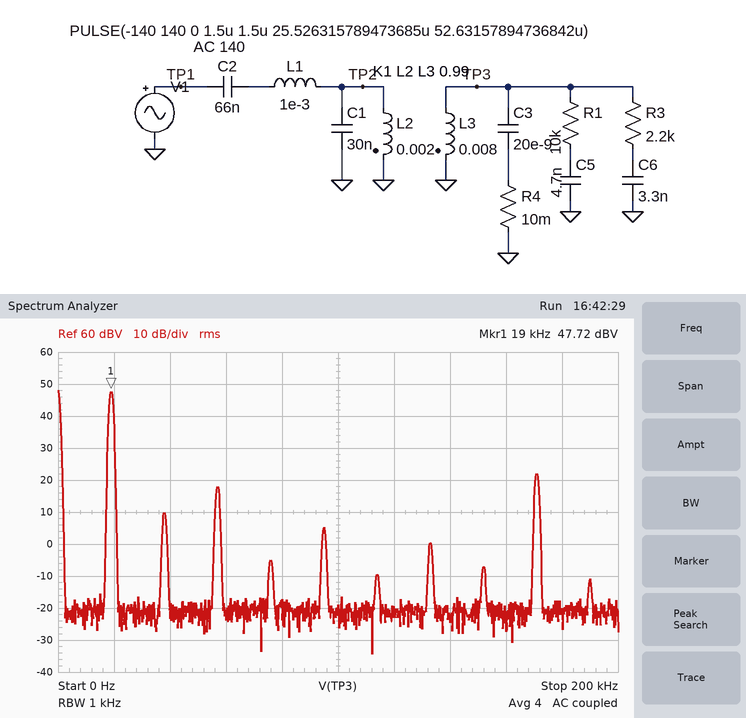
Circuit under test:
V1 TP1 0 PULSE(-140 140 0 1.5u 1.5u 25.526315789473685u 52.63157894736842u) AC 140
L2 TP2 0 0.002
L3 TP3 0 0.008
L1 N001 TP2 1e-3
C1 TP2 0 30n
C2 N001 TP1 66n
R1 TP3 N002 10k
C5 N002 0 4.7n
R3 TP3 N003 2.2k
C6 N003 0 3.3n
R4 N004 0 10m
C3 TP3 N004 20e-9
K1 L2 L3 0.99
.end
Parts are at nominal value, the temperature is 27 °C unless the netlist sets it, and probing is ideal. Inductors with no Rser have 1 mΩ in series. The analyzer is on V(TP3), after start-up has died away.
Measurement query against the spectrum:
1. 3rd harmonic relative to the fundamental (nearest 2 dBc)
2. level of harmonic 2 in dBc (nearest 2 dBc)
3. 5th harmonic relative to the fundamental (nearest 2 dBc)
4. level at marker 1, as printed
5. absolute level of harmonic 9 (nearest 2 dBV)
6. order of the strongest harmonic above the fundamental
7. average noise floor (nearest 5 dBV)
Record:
-30 dBc
-38 dBc
-42 dBc
47.72 dBV
22 dBV
9
-20 dBV
